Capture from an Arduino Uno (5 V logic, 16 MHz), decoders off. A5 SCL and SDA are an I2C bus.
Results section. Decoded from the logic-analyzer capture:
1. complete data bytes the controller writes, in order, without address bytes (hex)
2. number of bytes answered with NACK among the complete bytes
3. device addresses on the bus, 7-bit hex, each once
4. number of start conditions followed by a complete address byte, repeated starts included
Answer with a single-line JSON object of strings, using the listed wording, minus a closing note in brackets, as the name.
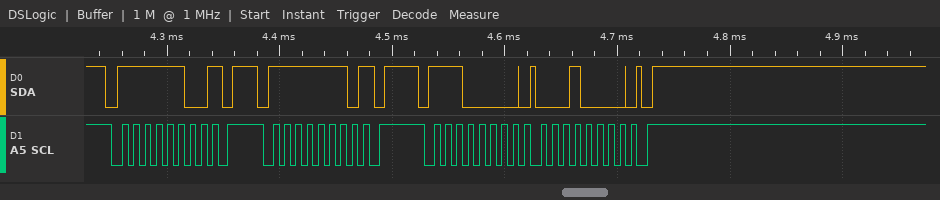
{"complete data bytes the controller writes, in order, without address bytes": "10", "number of bytes answered with NACK among the complete bytes": "2", "device addresses on the bus, 7-bit hex, each once": "0x7E 0x7F 0x70", "number of start conditions followed by a complete address byte, repeated starts included": "3"}
